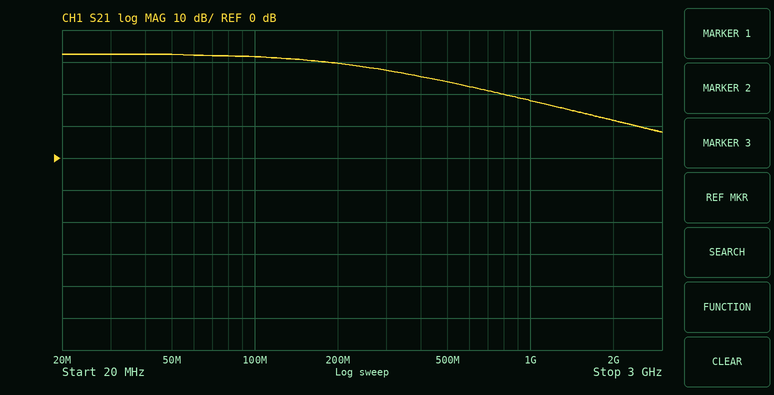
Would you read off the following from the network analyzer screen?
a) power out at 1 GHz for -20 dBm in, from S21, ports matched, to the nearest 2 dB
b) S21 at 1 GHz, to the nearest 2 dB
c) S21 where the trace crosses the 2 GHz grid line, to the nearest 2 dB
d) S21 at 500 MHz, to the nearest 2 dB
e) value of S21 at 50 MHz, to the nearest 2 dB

-2 dBm
18 dB
12 dB
24 dB
32 dB
